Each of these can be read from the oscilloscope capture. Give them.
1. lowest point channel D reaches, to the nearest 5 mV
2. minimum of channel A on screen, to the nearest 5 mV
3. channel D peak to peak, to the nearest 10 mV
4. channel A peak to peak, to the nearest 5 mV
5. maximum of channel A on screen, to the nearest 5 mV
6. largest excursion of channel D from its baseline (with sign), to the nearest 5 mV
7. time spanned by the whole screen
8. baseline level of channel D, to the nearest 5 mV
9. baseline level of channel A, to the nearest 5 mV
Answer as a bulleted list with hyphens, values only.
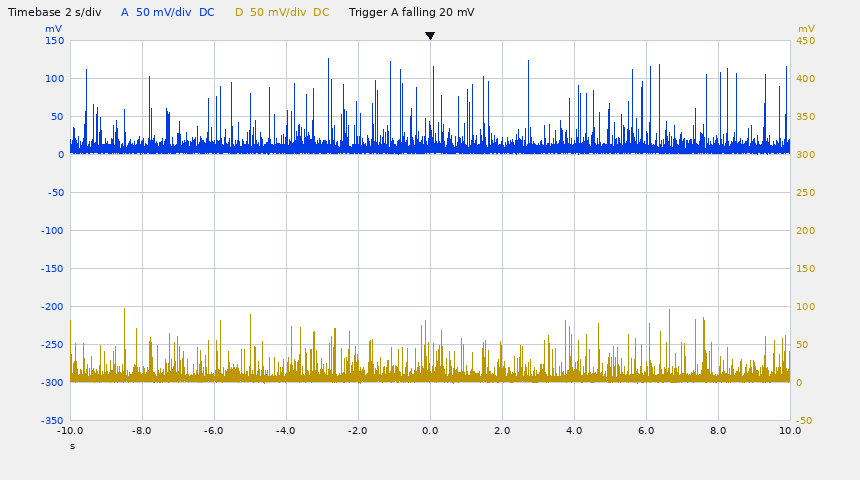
- 0 mV
- 0 mV
- 100 mV
- 125 mV
- 125 mV
- +90 mV
- 20 s
- 10 mV
- 10 mV
